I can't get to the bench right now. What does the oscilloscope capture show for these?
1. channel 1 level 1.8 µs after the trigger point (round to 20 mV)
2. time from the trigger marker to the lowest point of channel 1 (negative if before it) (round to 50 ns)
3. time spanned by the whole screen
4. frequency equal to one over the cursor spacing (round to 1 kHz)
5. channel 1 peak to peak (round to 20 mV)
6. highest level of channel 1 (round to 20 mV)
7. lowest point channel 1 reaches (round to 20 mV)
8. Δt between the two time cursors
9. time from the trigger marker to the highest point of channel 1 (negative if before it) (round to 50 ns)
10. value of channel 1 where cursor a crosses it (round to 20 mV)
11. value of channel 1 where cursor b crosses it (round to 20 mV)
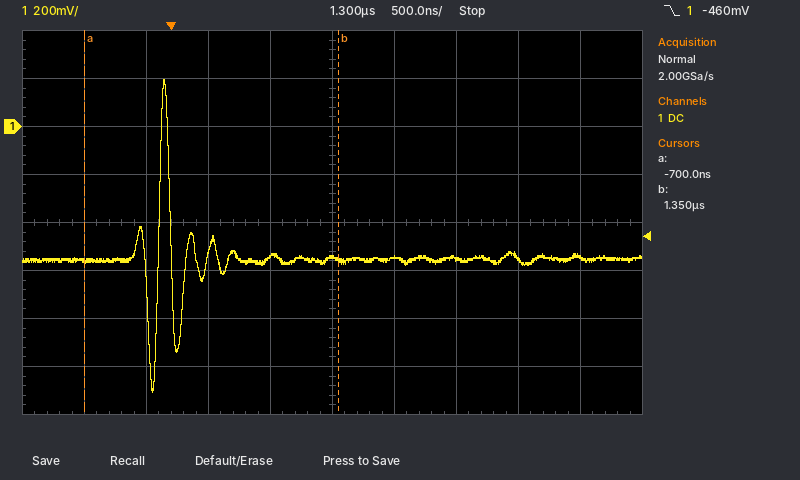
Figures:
-540 mV
-150 ns
5 µs
488 kHz
1.30 V
200 mV
-1.10 V
2.05 µs
-50 ns
-560 mV
-560 mV
